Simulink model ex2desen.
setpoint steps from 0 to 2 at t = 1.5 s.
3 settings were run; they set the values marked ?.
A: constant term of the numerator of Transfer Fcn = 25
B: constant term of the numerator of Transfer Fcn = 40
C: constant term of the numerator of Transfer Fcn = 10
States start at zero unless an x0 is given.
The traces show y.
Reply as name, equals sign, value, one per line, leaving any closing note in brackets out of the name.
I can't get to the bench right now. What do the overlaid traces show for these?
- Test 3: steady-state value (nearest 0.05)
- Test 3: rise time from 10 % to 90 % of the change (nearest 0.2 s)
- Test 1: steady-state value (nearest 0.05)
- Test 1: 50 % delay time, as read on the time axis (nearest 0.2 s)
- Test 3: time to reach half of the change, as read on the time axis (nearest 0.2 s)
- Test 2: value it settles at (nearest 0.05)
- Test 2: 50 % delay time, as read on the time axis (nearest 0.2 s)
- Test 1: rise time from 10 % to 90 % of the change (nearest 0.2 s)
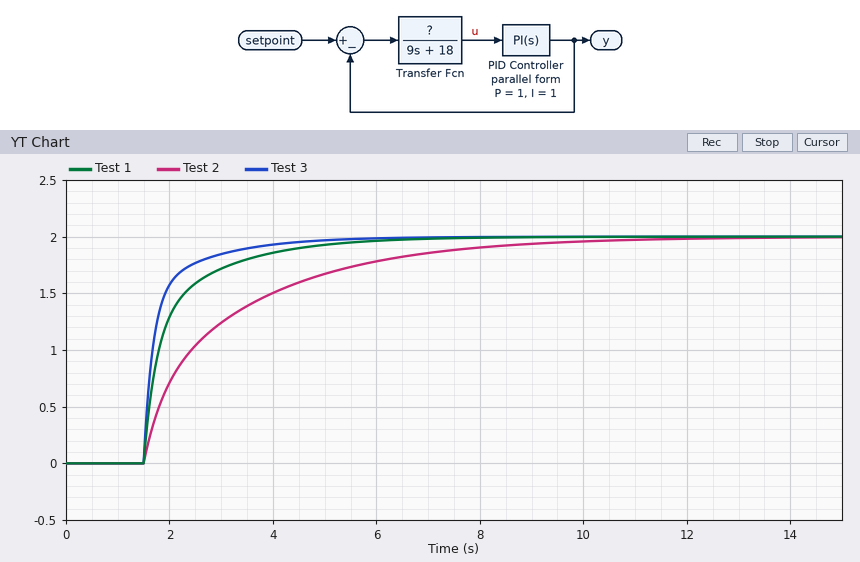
Test 3: steady-state value = 2.00
Test 3: rise time from 10 % to 90 % of the change = 1.2 s
Test 1: steady-state value = 2.00
Test 1: 50 % delay time, as read on the time axis = 1.8 s
Test 3: time to reach half of the change, as read on the time axis = 1.6 s
Test 2: value it settles at = 2.00
Test 2: 50 % delay time, as read on the time axis = 2.4 s
Test 1: rise time from 10 % to 90 % of the change = 2.0 s
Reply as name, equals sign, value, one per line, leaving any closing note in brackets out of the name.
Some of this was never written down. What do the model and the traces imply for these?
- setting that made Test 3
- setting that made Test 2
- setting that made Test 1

setting that made Test 3 = B
setting that made Test 2 = C
setting that made Test 1 = A
